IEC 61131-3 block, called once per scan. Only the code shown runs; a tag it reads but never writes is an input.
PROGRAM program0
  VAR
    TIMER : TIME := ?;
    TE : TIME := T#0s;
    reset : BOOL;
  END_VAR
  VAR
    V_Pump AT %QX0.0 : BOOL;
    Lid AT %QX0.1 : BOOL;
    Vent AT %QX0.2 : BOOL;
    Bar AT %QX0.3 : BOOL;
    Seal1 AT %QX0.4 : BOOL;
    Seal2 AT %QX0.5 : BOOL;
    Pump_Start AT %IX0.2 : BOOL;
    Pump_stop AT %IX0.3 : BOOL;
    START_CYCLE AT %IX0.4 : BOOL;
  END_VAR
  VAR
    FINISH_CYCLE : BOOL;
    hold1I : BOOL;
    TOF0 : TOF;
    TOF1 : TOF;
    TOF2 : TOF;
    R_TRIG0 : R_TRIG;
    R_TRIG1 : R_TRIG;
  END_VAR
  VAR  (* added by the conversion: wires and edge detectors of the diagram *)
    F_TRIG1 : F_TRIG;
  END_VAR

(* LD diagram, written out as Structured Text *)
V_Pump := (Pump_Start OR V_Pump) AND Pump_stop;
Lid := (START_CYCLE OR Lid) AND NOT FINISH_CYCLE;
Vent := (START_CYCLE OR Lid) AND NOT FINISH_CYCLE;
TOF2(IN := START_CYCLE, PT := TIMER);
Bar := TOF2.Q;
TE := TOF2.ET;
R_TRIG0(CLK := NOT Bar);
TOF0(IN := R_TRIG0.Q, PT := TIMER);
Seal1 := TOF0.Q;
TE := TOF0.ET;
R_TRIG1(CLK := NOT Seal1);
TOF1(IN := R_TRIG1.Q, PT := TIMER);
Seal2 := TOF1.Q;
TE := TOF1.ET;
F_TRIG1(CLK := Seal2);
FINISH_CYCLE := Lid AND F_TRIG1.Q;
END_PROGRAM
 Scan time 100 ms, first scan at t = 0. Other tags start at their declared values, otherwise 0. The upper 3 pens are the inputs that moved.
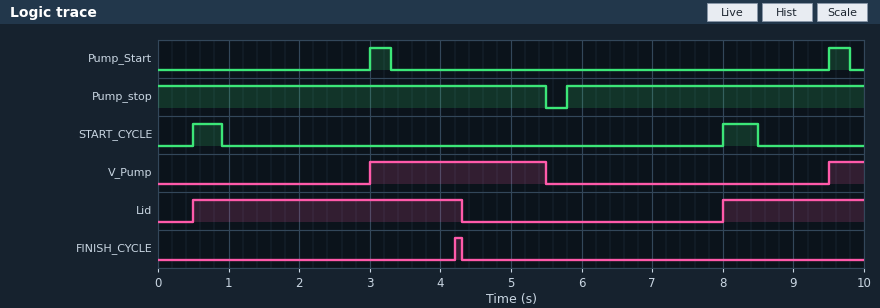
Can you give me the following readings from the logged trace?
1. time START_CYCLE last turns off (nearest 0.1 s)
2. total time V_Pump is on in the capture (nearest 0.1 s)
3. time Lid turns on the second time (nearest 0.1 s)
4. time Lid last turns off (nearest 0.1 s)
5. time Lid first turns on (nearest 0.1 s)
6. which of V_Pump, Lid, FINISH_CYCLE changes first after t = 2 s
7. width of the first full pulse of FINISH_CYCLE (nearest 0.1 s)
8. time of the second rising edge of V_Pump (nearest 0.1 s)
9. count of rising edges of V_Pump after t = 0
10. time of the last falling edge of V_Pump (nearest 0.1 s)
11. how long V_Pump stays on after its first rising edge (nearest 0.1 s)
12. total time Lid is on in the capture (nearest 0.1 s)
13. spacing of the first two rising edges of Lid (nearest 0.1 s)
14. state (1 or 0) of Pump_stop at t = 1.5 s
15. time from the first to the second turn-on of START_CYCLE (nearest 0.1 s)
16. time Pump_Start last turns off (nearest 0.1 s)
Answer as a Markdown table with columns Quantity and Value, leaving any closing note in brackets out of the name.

| Quantity | Value |
|---|---|
| time START_CYCLE last turns off | 8.5 s |
| total time V_Pump is on in the capture | 3.0 s |
| time Lid turns on the second time | 8.0 s |
| time Lid last turns off | 4.3 s |
| time Lid first turns on | 0.5 s |
| which of V_Pump, Lid, FINISH_CYCLE changes first after t = 2 s | V_Pump |
| width of the first full pulse of FINISH_CYCLE | 0.1 s |
| time of the second rising edge of V_Pump | 9.5 s |
| count of rising edges of V_Pump after t = 0 | 2 |
| time of the last falling edge of V_Pump | 5.5 s |
| how long V_Pump stays on after its first rising edge | 2.5 s |
| total time Lid is on in the capture | 5.8 s |
| spacing of the first two rising edges of Lid | 7.5 s |
| state (1 or 0) of Pump_stop at t = 1.5 s | 1 |
| time from the first to the second turn-on of START_CYCLE | 7.5 s |
| time Pump_Start last turns off | 9.8 s |
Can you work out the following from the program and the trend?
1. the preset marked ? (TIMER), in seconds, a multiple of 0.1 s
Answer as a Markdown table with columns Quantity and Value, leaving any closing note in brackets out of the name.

| Quantity | Value |
|---|---|
| the preset marked ? (TIMER), in seconds, a multiple of 0.1 s | 2.0 s |
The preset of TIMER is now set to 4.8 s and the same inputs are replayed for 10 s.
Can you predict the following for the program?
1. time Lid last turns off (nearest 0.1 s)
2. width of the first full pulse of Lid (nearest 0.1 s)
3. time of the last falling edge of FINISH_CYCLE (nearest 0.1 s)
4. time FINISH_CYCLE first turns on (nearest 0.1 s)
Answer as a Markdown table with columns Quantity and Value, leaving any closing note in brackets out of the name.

| Quantity | Value |
|---|---|
| time Lid last turns off | 9.9 s |
| width of the first full pulse of Lid | 9.4 s |
| time of the last falling edge of FINISH_CYCLE | 9.9 s |
| time FINISH_CYCLE first turns on | 9.8 s |
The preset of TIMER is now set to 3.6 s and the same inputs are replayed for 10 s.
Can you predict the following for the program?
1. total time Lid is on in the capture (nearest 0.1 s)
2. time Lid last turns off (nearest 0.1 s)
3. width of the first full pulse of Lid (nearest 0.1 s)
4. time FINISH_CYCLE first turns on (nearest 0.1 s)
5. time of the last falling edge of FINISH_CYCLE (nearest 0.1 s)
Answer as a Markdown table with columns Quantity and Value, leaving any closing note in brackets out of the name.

| Quantity | Value |
|---|---|
| total time Lid is on in the capture | 9.0 s |
| time Lid last turns off | 7.5 s |
| width of the first full pulse of Lid | 7.0 s |
| time FINISH_CYCLE first turns on | 7.4 s |
| time of the last falling edge of FINISH_CYCLE | 7.5 s |
